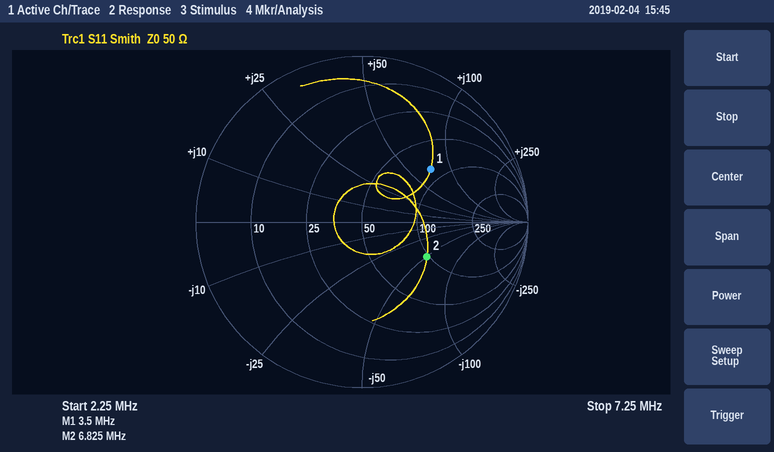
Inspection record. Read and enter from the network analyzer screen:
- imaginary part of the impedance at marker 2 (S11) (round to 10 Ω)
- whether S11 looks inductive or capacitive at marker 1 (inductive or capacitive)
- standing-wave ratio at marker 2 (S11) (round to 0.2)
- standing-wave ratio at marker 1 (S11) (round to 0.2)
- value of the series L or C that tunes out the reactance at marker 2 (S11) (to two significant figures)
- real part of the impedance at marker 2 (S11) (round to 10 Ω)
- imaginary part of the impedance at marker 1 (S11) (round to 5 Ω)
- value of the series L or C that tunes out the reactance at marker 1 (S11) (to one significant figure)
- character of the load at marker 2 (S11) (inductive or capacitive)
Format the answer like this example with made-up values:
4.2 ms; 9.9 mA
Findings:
-50 Ω; inductive; 2.6; 3.2; 1.2 µH; 100 Ω; +70 Ω; 600 pF; capacitive
